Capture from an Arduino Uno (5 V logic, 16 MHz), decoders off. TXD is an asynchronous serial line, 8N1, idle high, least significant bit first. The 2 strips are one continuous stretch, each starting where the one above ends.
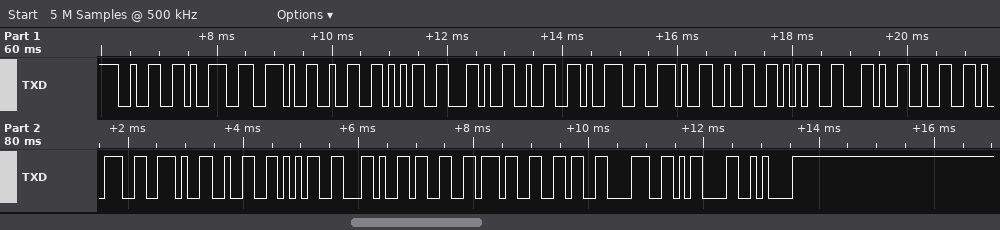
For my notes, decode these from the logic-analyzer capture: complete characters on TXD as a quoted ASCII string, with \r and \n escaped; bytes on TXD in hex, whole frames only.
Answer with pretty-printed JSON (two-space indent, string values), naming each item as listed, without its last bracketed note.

{
  "complete characters on TXD as a quoted ASCII string, with \\r and \\n escaped": "\"29.25,29.25,29.25,3768\\r\\n\"",
  "bytes on TXD in hex, whole frames only": "32 39 2E 32 35 2C 32 39 2E 32 35 2C 32 39 2E 32 35 2C 33 37 36 38 0D 0A"
}
